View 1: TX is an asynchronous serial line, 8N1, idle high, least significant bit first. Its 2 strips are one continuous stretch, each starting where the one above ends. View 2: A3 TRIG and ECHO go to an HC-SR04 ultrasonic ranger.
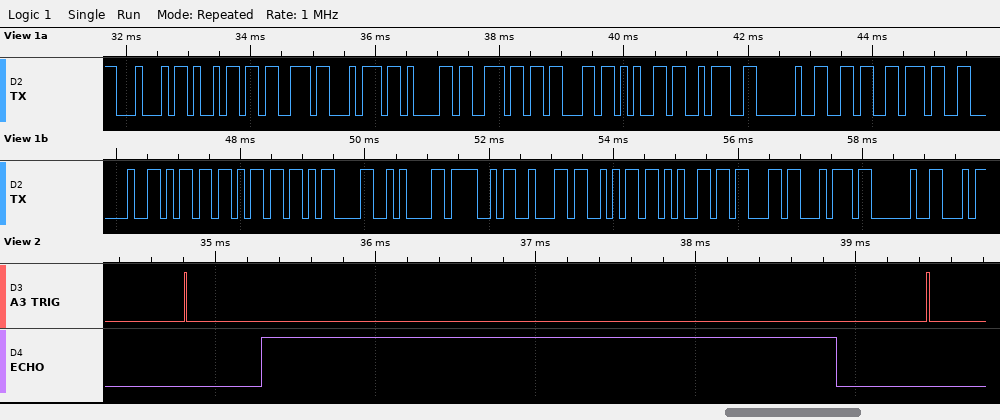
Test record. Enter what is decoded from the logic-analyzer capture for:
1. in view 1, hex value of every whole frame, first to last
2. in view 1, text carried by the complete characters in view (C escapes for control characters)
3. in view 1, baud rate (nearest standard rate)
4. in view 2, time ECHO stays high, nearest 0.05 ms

0x44 0x69 0x73 0x74 0x61 0x6E 0x63 0x65 0x3A 0x20 0x36 0x37 0x20 0x6D 0x6D 0x0D 0x0A 0x4F 0x62 0x6A 0x65 0x63 0x74 0x20
"Distance: 67 mm\r\nObject "
9600 baud
3.60 ms
